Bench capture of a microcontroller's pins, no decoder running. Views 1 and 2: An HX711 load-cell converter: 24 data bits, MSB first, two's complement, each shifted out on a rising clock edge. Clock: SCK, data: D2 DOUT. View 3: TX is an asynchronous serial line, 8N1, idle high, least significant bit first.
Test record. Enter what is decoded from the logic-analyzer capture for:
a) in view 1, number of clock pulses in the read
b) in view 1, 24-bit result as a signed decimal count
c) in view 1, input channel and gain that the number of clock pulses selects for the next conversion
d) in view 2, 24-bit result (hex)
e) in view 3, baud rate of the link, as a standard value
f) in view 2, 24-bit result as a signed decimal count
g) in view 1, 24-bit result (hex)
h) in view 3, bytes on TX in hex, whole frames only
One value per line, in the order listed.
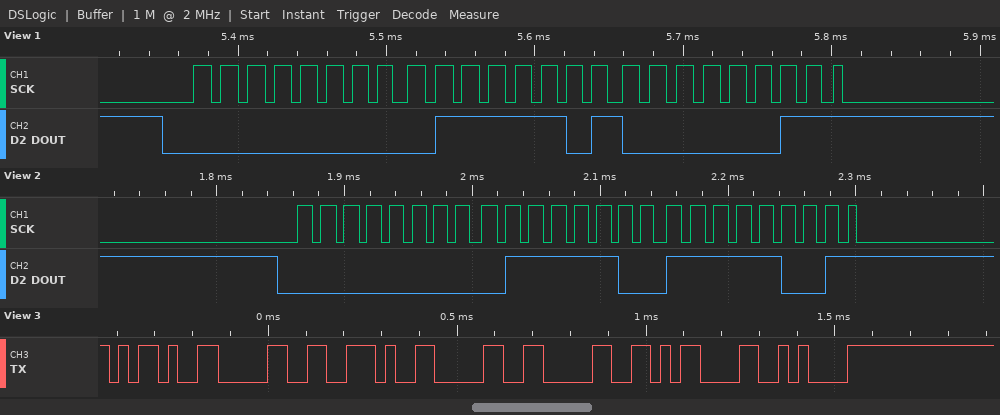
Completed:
25
32003
channel A, gain 128
0x007CF9
38400 baud
31993
0x007D03
0x2D 0x30 0x2E 0x30 0x30 0x0D 0x0A
